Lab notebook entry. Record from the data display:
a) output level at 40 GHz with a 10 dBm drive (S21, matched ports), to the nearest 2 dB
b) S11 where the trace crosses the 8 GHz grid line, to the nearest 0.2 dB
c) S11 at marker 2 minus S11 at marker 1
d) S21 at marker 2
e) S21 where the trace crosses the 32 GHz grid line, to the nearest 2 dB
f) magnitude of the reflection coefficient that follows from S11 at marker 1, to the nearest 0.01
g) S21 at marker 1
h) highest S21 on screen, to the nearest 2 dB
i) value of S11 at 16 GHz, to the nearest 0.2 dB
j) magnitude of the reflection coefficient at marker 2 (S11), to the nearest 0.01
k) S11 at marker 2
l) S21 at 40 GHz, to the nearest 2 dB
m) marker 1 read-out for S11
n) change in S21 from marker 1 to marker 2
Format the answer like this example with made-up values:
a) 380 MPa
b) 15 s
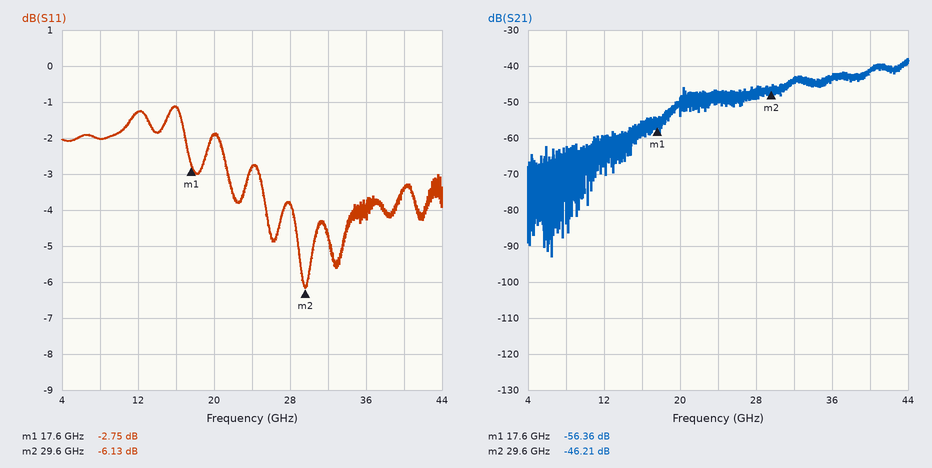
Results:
a) -32 dBm
b) -2.0 dB
c) -3.38 dB
d) -46.21 dB
e) -44 dB
f) 0.73
g) -56.36 dB
h) -38 dB
i) -1.2 dB
j) 0.49
k) -6.13 dB
l) -42 dB
m) -2.75 dB
n) 10.15 dB
